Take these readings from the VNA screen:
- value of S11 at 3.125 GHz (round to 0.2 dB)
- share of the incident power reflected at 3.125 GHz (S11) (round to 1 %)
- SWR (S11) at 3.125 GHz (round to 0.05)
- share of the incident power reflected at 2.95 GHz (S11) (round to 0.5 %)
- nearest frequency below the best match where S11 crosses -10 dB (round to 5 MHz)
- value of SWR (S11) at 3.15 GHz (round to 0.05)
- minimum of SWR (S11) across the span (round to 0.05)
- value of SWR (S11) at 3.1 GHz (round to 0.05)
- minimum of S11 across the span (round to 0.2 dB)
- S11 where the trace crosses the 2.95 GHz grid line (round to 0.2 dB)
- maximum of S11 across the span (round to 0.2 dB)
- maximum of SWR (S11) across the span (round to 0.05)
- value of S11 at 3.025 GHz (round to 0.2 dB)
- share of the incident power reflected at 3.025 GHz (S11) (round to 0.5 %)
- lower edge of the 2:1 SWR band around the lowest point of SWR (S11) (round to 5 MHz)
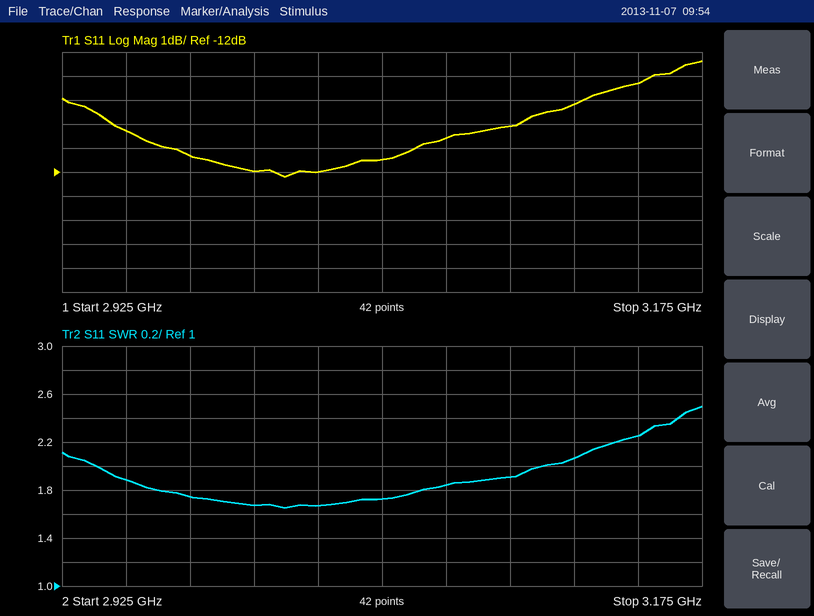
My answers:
-9.2 dB
12 %
2.05
9.5 %
2.945 GHz
2.25
1.65
1.90
-12.2 dB
-10.2 dB
-7.4 dB
2.50
-12.0 dB
6.5 %
2.940 GHz
